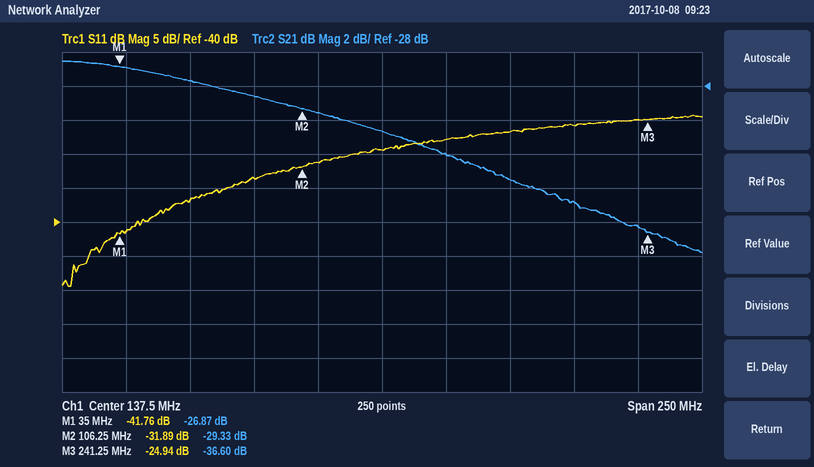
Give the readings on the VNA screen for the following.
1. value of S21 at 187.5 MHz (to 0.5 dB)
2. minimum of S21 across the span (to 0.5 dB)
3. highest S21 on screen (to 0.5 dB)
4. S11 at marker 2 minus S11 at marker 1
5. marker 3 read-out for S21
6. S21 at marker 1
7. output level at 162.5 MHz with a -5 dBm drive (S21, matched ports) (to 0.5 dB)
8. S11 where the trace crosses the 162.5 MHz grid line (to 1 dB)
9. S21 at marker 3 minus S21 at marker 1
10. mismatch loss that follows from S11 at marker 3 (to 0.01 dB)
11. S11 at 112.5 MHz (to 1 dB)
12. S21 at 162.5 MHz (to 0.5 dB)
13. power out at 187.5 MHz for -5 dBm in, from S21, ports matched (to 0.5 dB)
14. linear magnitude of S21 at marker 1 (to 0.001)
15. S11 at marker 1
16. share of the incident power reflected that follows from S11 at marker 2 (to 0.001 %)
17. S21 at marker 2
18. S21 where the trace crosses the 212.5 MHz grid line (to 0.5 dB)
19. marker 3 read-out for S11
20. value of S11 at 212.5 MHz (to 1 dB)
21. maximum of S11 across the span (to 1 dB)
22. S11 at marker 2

-33.5 dB
-38.0 dB
-26.5 dB
9.87 dB
-36.60 dB
-26.87 dB
-37.0 dBm
-28 dB
-9.73 dB
0.01 dB
-31 dB
-32.0 dB
-38.5 dBm
0.045
-41.76 dB
0.065 %
-29.33 dB
-35.0 dB
-24.94 dB
-26 dB
-24 dB
-31.89 dB
